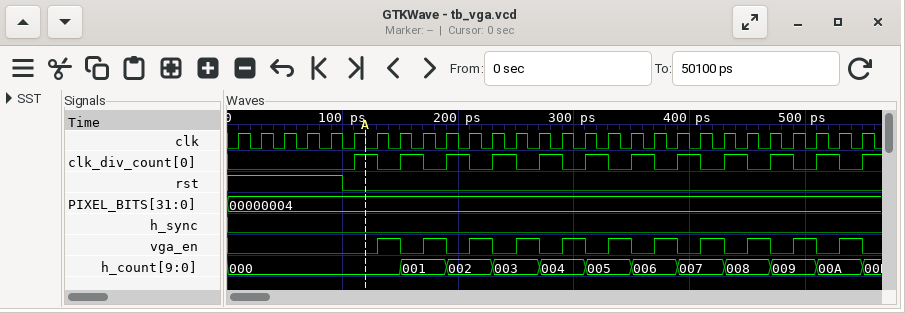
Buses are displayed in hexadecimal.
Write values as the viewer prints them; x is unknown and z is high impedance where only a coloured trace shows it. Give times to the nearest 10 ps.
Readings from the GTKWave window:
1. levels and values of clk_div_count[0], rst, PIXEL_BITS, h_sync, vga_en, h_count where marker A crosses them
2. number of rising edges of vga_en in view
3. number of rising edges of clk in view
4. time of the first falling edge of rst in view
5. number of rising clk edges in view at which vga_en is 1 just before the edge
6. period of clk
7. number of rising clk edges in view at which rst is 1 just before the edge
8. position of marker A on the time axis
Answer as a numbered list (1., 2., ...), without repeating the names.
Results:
1. clk_div_count[0]=1, rst=0, PIXEL_BITS=00000004, h_sync=0, vga_en=0, h_count=000
2. 11
3. 28
4. 100 ps
5. 11
6. 20 ps
7. 5
8. 120 ps
